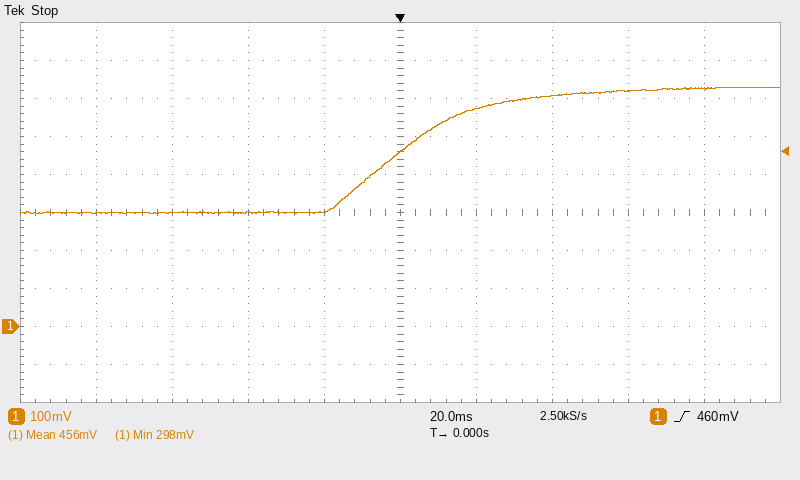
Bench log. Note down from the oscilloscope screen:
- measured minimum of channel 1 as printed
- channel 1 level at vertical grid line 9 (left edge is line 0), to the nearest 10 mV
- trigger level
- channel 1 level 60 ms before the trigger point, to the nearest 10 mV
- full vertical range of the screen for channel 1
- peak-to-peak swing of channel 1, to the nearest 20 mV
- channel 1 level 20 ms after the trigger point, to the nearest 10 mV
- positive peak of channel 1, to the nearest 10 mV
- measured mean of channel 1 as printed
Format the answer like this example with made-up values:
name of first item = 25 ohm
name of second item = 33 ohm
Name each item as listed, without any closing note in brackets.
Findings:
measured minimum of channel 1 as printed = 298 mV
channel 1 level at vertical grid line 9 (left edge is line 0), to the nearest 10 mV = 630 mV
trigger level = 460 mV
channel 1 level 60 ms before the trigger point, to the nearest 10 mV = 300 mV
full vertical range of the screen for channel 1 = 1 V
peak-to-peak swing of channel 1, to the nearest 20 mV = 340 mV
channel 1 level 20 ms after the trigger point, to the nearest 10 mV = 570 mV
positive peak of channel 1, to the nearest 10 mV = 630 mV
measured mean of channel 1 as printed = 456 mV
